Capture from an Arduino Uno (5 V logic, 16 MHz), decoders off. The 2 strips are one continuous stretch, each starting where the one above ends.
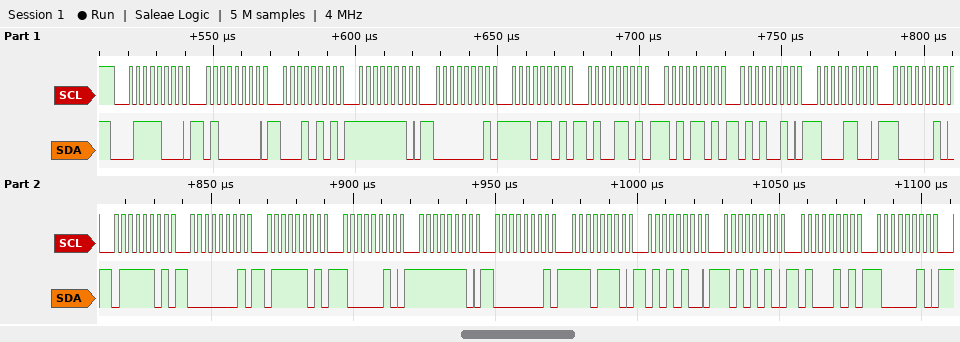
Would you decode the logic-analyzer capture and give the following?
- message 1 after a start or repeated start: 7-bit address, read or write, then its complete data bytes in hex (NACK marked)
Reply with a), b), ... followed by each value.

a) 0x3C write: 40 15 FE 01 ED 4D AD 52 8C 82 7D 01 7D 82 FE 01 EE 54 AA 45 82
